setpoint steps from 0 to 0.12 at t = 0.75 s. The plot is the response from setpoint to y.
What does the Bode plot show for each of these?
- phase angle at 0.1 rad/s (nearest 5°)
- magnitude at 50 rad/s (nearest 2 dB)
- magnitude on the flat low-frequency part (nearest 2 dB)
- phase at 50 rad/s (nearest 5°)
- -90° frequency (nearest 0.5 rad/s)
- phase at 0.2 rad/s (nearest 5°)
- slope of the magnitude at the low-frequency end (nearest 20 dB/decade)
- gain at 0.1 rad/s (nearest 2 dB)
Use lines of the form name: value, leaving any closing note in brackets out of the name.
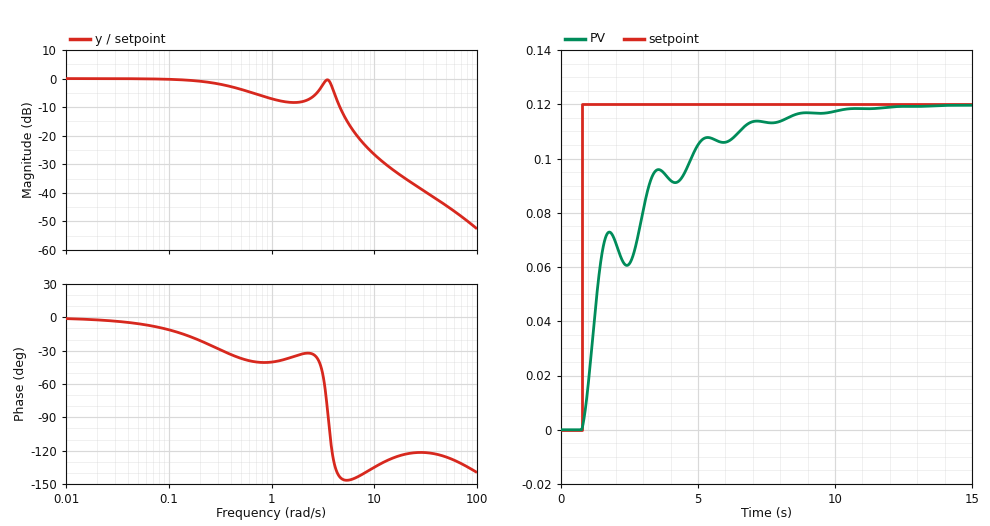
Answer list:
phase angle at 0.1 rad/s: -10°
magnitude at 50 rad/s: -44 dB
magnitude on the flat low-frequency part: 0 dB
phase at 50 rad/s: -125°
-90° frequency: 3.5 rad/s
phase at 0.2 rad/s: -20°
slope of the magnitude at the low-frequency end: 0 dB/decade
gain at 0.1 rad/s: 0 dB
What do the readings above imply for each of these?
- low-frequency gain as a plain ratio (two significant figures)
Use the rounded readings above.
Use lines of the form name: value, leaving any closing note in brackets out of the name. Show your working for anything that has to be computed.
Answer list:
low-frequency gain as a plain ratio: 10^(0 / 20) = 1.0
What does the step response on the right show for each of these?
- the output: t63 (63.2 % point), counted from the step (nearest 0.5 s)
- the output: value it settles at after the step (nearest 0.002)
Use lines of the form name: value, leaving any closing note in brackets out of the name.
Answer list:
the output: t63 (63.2 % point), counted from the step: 2.0 s
the output: value it settles at after the step: 0.120
